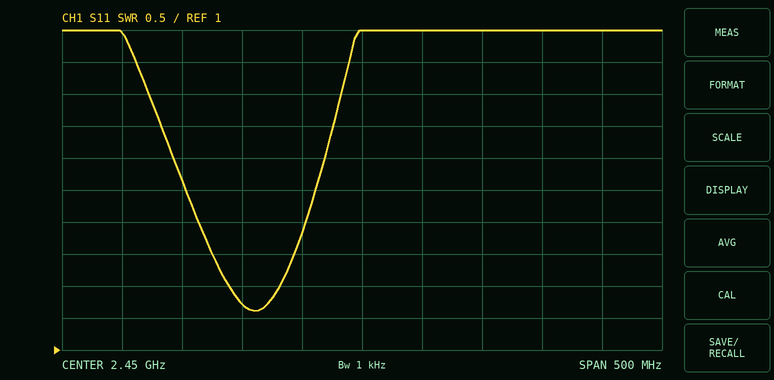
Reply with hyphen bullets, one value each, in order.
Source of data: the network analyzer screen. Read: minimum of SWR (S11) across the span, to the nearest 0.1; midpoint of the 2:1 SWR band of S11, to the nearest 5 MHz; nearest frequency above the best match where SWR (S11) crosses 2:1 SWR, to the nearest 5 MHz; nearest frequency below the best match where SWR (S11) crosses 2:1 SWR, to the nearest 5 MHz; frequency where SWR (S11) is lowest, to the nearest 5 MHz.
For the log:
- 1.6
- 2.360 GHz
- 2.380 GHz
- 2.340 GHz
- 2.360 GHz
